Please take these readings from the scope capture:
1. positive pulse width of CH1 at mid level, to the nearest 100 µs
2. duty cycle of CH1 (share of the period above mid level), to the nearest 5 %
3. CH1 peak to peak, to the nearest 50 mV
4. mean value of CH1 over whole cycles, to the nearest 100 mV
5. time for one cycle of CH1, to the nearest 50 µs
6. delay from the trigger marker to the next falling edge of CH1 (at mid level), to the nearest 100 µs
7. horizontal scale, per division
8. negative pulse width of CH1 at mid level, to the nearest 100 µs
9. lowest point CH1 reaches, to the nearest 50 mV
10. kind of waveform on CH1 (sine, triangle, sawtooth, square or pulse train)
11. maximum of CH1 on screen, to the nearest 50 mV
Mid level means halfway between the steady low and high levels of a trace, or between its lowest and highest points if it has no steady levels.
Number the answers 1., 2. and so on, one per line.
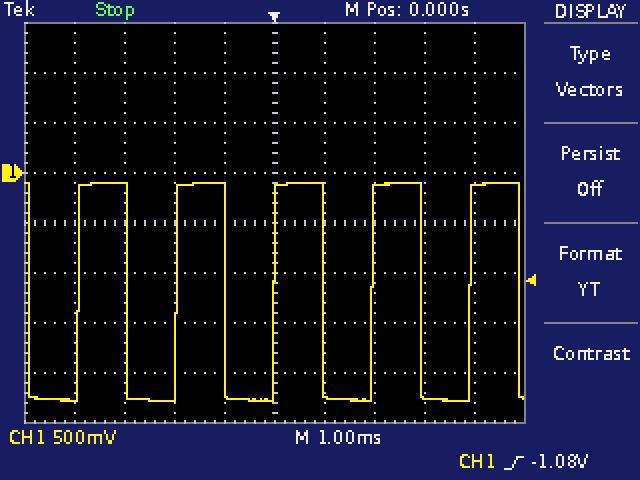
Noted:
1. 1.0 ms
2. 50 %
3. 2.20 V
4. -1.2 V
5. 1.95 ms
6. 1.0 ms
7. 1 ms
8. 1.0 ms
9. -2.30 V
10. square
11. -100 mV
